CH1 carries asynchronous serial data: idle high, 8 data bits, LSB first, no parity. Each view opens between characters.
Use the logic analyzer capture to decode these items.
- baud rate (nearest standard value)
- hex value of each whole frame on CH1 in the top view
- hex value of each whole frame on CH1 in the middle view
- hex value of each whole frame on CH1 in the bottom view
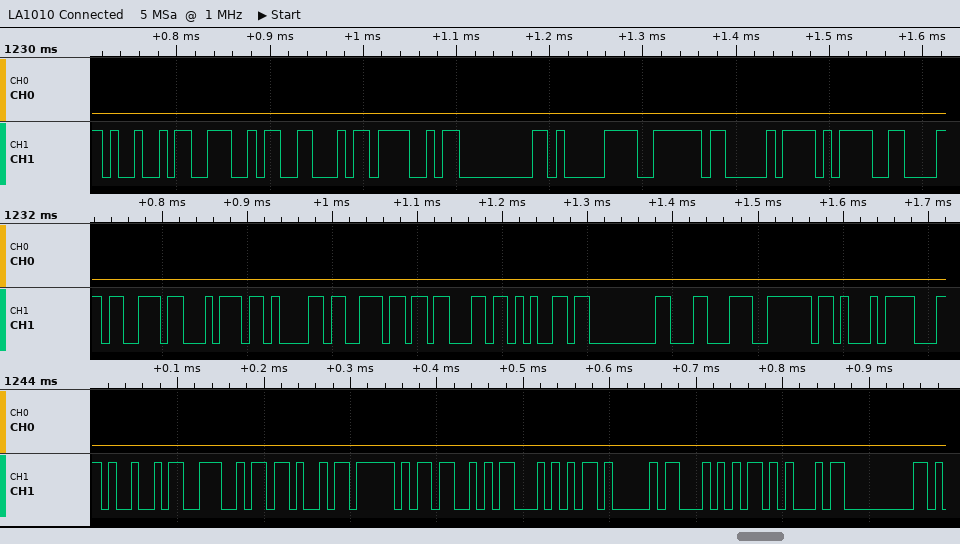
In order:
115200 baud
49, 4E, 46, 4F, 00, C1, 7E, D0, 3D
73, 74, 61, 6E, 63, 65, 00, 8C, 7E, D1
49, 4E, 4B, 5F, 53, 54, 41, 54, 45, 00
